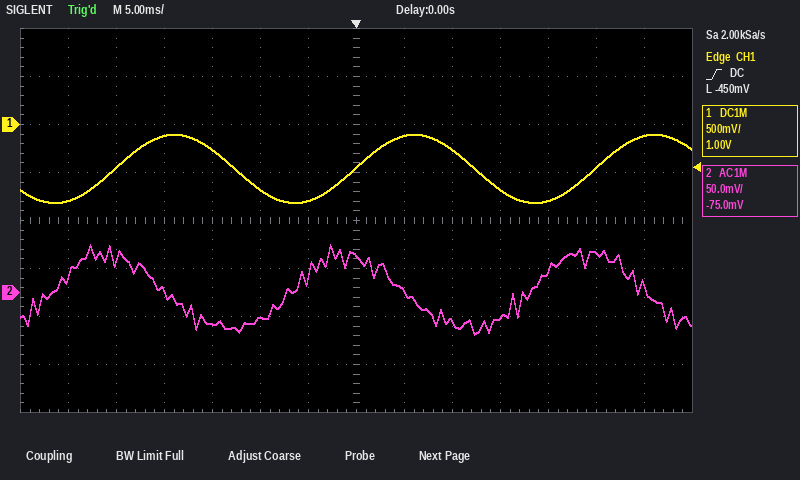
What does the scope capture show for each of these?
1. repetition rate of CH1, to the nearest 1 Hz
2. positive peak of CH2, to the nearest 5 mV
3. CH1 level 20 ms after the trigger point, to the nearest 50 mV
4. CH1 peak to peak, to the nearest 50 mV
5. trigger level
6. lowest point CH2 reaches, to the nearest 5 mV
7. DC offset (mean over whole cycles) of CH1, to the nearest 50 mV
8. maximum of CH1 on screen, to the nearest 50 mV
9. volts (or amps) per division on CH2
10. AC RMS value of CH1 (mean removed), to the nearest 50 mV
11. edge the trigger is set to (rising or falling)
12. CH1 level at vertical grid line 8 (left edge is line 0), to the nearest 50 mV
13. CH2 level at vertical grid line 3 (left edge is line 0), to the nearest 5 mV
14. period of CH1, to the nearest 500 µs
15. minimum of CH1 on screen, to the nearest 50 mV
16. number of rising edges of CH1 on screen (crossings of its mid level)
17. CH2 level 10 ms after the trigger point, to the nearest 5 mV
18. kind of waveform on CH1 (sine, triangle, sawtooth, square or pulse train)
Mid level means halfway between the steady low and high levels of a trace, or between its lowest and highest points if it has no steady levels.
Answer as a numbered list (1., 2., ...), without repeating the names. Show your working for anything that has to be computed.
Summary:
1. 1 / 25.0 ms ≈ 40 Hz
2. 50 mV
3. -800 mV
4. -100 mV − (-800 mV) = 700 mV
5. -450 mV
6. -45 mV
7. (-100 mV + (-800 mV)) / 2 ≈ -450 mV
8. -100 mV
9. 50 mV
10. 700 mV / (2√2) ≈ 247 mV, so 250 mV to the nearest 50 mV
11. rising
12. -100 mV
13. 0 mV
14. 25.0 ms
15. -800 mV
16. 3
17. -30 mV
18. sine
